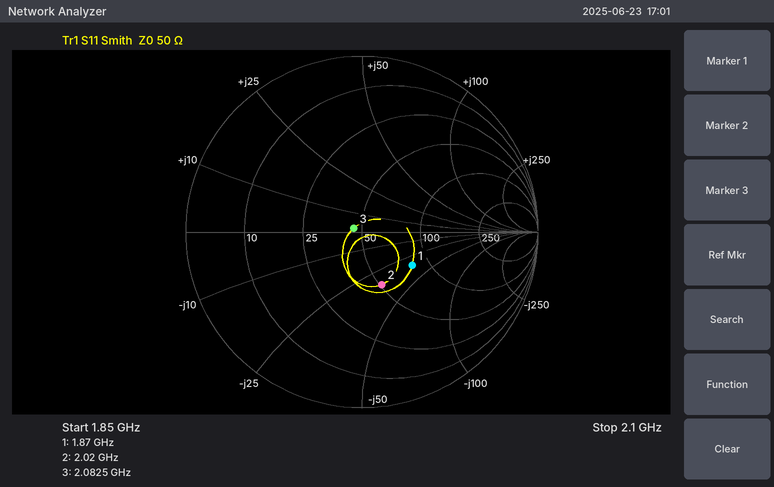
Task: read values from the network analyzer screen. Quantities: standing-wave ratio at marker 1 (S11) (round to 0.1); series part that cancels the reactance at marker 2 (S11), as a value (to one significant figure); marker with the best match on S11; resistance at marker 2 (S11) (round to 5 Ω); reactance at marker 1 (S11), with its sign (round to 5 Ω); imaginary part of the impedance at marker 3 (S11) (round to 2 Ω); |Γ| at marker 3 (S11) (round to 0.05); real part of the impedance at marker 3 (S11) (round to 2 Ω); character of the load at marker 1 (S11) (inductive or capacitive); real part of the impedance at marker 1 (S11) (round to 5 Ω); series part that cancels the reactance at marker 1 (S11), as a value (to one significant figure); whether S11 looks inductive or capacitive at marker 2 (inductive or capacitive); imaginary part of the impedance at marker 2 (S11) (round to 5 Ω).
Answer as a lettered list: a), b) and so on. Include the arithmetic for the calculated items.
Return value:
a) 2.0
b) L = 35 Ω/(2π × 2.02 GHz) ≈ 3 nH
c) marker 3
d) 50 Ω
e) -35 Ω
f) +2 Ω
g) 0.05
h) 46 Ω
i) capacitive
j) 80 Ω
k) L = 35 Ω/(2π × 1.87 GHz) ≈ 3 nH
l) capacitive
m) -35 Ω
